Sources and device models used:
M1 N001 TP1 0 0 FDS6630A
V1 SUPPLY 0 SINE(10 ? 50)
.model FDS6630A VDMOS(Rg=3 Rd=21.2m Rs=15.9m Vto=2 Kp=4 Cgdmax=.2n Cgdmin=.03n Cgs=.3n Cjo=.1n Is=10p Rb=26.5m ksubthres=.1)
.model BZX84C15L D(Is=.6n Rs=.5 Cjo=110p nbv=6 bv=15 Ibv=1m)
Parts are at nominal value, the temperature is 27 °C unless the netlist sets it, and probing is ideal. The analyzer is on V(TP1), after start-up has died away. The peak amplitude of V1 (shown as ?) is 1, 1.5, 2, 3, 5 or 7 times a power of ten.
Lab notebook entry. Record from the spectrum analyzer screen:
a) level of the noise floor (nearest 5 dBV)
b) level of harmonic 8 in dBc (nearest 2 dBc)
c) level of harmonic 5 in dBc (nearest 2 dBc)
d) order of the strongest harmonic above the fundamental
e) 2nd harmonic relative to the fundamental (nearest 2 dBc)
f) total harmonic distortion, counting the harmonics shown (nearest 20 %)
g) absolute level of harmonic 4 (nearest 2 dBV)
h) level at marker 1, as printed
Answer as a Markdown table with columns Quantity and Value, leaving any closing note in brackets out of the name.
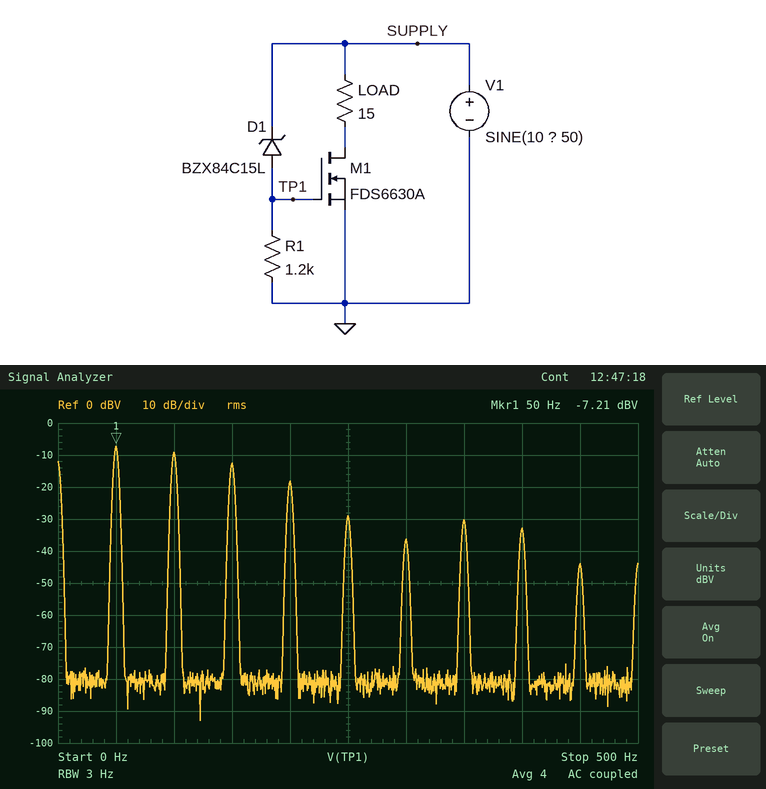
| Quantity | Value |
|---|---|
| level of the noise floor | -80 dBV |
| level of harmonic 8 in dBc | -26 dBc |
| level of harmonic 5 in dBc | -22 dBc |
| order of the strongest harmonic above the fundamental | 2 |
| 2nd harmonic relative to the fundamental | -2 dBc |
| total harmonic distortion, counting the harmonics shown | 100 % |
| absolute level of harmonic 4 | -18 dBV |
| level at marker 1, as printed | -7.21 dBV |
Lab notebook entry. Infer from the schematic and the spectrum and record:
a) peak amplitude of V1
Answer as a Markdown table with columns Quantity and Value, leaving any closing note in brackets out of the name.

| Quantity | Value |
|---|---|
| peak amplitude of V1 | 7 V |
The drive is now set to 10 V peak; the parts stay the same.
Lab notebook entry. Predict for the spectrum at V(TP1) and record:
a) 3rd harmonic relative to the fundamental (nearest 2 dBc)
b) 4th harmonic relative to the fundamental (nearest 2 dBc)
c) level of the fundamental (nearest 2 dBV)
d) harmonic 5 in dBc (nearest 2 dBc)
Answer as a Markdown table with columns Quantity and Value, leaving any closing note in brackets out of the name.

| Quantity | Value |
|---|---|
| 3rd harmonic relative to the fundamental | -10 dBc |
| 4th harmonic relative to the fundamental | -24 dBc |
| level of the fundamental | 2 dBV |
| harmonic 5 in dBc | -24 dBc |
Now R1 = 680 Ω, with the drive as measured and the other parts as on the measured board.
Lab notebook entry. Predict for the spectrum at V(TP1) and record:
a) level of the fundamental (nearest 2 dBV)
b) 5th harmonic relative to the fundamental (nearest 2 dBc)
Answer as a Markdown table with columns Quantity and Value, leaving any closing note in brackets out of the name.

| Quantity | Value |
|---|---|
| level of the fundamental | -8 dBV |
| 5th harmonic relative to the fundamental | -20 dBc |
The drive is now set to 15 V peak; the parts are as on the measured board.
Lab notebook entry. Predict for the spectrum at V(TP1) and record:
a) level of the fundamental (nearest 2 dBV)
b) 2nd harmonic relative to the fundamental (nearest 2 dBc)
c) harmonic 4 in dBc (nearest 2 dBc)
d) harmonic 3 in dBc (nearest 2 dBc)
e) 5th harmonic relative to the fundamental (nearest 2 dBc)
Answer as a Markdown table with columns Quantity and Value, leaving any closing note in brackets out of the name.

| Quantity | Value |
|---|---|
| level of the fundamental | 12 dBV |
| 2nd harmonic relative to the fundamental | -12 dBc |
| harmonic 4 in dBc | -20 dBc |
| harmonic 3 in dBc | -10 dBc |
| 5th harmonic relative to the fundamental | -28 dBc |
